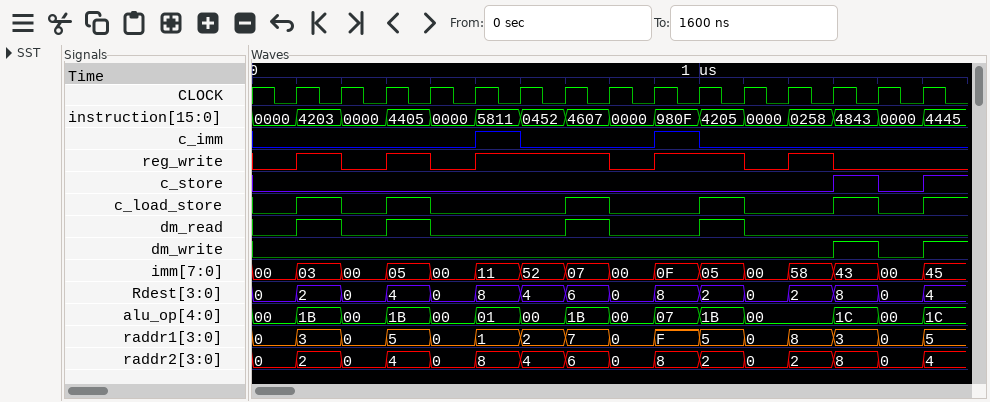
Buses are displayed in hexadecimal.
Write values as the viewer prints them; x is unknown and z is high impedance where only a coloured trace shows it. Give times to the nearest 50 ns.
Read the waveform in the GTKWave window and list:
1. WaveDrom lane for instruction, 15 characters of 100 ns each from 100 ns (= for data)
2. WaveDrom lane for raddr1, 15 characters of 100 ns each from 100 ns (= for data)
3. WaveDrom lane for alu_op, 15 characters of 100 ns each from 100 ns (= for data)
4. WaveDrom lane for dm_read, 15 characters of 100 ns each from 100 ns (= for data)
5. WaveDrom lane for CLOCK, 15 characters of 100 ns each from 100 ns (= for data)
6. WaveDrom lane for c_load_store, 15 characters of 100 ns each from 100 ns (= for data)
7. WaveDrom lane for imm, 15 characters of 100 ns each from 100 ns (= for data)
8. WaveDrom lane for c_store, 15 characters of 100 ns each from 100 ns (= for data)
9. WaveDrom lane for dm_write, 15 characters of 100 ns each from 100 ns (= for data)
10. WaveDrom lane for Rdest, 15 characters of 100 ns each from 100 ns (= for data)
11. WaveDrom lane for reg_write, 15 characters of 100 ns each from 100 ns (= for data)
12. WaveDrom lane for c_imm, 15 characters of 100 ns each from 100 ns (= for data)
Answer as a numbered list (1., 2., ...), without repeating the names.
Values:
1. {name: 'instruction', wave: '===============', data: '4203 0000 4405 0000 5811 0452 4607 0000 980F 4205 0000 0258 4843 0000 4445'}
2. {name: 'raddr1', wave: '===============', data: '3 0 5 0 1 2 7 0 F 5 0 8 3 0 5'}
3. {name: 'alu_op', wave: '===========.===', data: '1B 00 1B 00 01 00 1B 00 07 1B 00 1C 00 1C'}
4. {name: 'dm_read', wave: '1010..10.10....'}
5. {name: 'CLOCK', wave: 'p..............'}
6. {name: 'c_load_store', wave: '1010..10.10.101'}
7. {name: 'imm', wave: '===============', data: '03 00 05 00 11 52 07 00 0F 05 00 58 43 00 45'}
8. {name: 'c_store', wave: '0...........101'}
9. {name: 'dm_write', wave: '0...........101'}
10. {name: 'Rdest', wave: '===============', data: '2 0 4 0 8 4 6 0 8 2 0 2 8 0 4'}
11. {name: 'reg_write', wave: '10101..01.010..'}
12. {name: 'c_imm', wave: '0...10..10.....'}
